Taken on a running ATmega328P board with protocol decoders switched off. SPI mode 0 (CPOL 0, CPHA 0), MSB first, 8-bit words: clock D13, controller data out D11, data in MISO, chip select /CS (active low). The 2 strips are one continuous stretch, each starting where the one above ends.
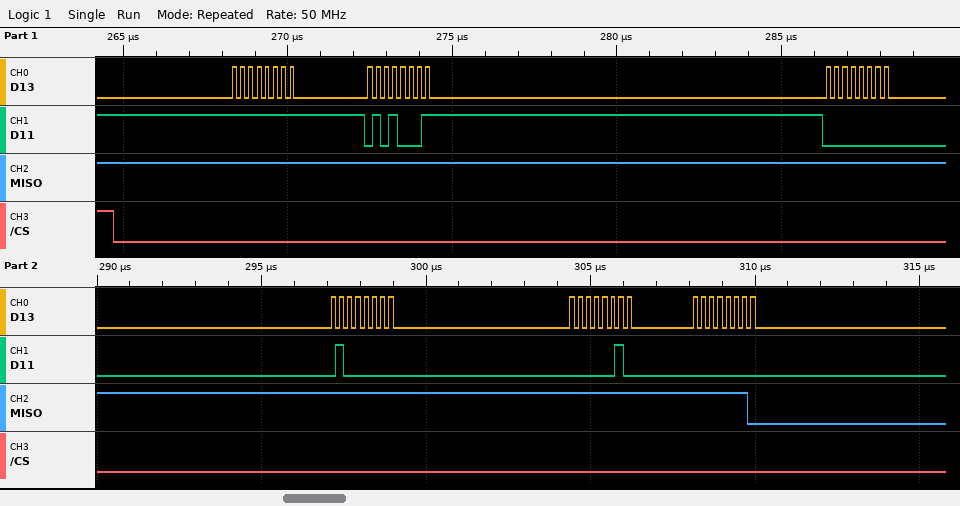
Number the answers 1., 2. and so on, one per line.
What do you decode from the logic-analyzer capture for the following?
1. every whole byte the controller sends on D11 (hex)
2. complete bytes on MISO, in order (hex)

1. FF 51 00 40 02 00
2. FF FF FF FF FF FE
